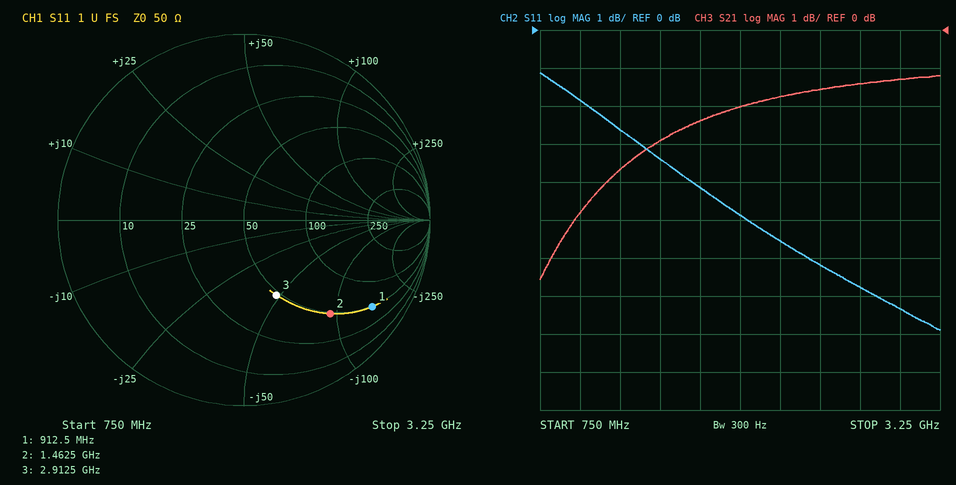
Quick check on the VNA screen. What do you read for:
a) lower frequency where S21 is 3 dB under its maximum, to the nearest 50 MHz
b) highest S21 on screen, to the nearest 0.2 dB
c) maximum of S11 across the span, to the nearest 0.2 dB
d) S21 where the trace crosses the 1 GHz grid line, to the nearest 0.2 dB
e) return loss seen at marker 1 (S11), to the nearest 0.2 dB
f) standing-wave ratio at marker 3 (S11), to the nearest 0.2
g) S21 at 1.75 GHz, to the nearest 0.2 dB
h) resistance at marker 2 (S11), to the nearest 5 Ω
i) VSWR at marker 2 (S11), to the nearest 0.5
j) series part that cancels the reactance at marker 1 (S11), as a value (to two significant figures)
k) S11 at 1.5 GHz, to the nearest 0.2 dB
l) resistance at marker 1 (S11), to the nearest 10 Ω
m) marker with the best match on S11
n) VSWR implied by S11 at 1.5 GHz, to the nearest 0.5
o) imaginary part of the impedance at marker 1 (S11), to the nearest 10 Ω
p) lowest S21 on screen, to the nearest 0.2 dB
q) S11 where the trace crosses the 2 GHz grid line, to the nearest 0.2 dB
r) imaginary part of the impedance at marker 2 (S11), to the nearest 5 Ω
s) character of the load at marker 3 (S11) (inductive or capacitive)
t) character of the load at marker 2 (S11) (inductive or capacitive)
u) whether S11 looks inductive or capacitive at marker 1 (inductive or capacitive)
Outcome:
1.10 GHz
-1.2 dB
-1.2 dB
-4.8 dB
1.6 dB
2.6
-2.4 dB
50 Ω
5.5
26 nH
-3.4 dB
50 Ω
marker 3
5.0
-150 Ω
-6.6 dB
-4.8 dB
-95 Ω
capacitive
capacitive
capacitive
